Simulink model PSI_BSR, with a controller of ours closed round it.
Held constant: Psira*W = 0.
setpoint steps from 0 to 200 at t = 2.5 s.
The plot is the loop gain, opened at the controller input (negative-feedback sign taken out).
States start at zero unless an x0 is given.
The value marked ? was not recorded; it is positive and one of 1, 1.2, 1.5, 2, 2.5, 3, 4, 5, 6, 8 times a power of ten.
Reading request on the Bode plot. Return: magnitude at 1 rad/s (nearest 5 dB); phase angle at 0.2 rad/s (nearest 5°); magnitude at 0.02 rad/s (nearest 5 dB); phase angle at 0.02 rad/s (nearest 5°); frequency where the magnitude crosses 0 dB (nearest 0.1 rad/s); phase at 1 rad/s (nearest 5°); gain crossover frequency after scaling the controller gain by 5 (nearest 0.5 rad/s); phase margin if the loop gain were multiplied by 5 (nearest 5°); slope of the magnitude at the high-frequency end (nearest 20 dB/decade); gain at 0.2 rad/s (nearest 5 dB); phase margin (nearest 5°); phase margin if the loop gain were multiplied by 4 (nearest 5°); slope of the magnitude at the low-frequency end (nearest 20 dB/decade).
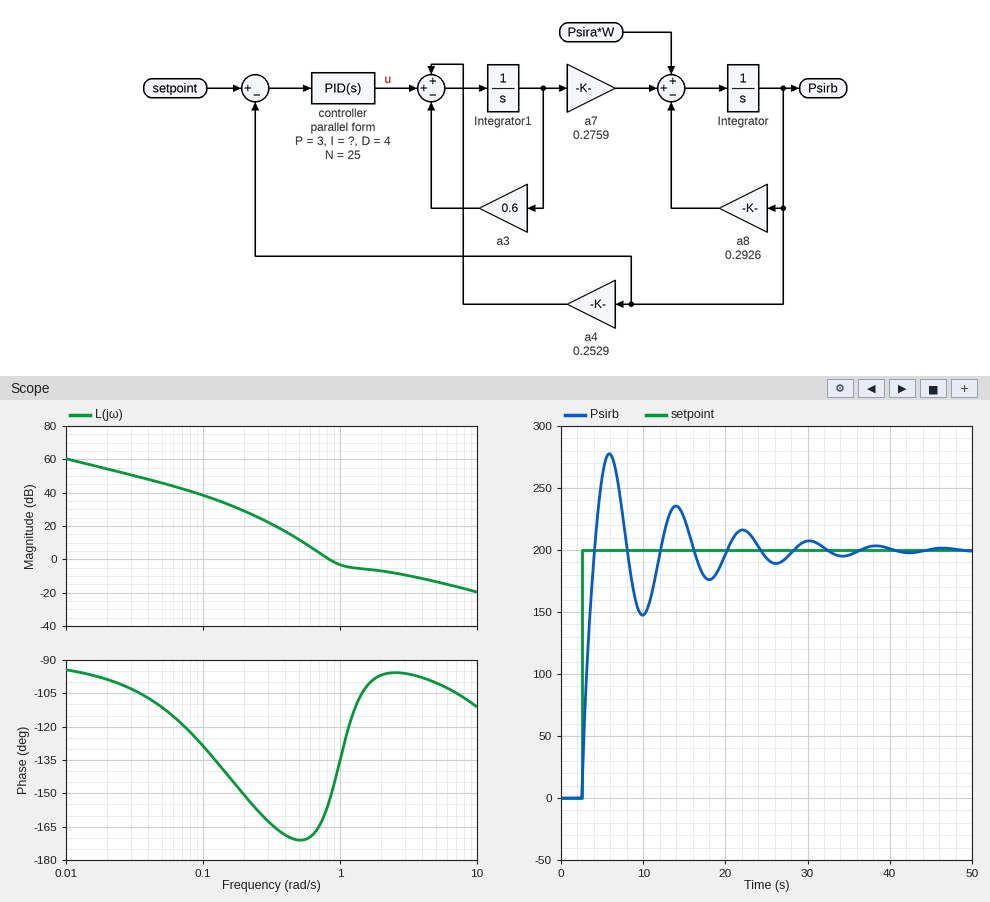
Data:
-5 dB
-150°
55 dB
-100°
0.8 rad/s
-135°
5.5 rad/s
80°
-20 dB/decade
30 dB
25°
80°
-20 dB/decade
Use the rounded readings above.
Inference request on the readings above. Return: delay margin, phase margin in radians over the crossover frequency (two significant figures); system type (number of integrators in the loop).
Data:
0.55 s
1
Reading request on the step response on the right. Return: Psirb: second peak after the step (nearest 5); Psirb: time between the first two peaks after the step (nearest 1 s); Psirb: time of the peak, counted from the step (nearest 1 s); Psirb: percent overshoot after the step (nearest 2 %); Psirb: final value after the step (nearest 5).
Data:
235
8 s
3 s
38 %
200
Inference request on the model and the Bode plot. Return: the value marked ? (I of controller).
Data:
4
